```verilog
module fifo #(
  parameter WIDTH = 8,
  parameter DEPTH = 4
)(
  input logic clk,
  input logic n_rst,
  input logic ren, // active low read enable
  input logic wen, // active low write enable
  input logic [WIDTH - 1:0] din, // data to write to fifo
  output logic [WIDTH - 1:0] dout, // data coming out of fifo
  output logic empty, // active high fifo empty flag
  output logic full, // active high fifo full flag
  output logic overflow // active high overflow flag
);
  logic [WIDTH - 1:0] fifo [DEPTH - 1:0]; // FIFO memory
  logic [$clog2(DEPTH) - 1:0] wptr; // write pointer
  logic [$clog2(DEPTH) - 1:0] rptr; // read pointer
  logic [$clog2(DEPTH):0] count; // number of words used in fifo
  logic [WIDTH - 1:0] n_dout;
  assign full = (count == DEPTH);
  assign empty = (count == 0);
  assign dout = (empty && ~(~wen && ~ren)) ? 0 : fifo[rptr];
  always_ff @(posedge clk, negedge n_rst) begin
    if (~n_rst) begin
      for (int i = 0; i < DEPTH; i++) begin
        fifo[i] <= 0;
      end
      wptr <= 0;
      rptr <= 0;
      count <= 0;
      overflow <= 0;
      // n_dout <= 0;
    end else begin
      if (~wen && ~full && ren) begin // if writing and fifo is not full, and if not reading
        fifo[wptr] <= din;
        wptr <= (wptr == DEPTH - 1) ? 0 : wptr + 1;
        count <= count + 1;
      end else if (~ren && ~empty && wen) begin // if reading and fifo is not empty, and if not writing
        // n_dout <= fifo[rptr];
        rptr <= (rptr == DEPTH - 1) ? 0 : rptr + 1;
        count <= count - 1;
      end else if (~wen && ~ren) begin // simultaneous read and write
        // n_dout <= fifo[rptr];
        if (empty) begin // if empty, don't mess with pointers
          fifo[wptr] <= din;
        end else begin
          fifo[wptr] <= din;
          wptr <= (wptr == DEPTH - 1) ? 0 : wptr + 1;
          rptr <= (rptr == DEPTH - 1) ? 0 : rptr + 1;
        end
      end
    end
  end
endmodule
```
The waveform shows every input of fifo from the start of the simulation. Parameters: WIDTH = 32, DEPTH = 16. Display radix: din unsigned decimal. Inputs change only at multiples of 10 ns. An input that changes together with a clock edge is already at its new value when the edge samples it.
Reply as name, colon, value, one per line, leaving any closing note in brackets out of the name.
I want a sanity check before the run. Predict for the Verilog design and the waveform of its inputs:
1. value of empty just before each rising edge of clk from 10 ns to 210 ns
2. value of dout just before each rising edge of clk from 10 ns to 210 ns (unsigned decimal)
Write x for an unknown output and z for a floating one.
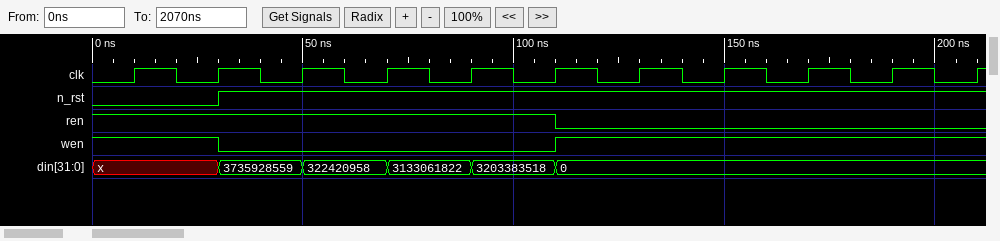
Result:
value of empty just before each rising edge of clk from 10 ns to 210 ns: 1 1 0 0 0 0 0 0 0 1 1
value of dout just before each rising edge of clk from 10 ns to 210 ns: 0, 0, 3735928559, 3735928559, 3735928559, 3735928559, 322420958, 3133061822, 3203383518, 0, 0
